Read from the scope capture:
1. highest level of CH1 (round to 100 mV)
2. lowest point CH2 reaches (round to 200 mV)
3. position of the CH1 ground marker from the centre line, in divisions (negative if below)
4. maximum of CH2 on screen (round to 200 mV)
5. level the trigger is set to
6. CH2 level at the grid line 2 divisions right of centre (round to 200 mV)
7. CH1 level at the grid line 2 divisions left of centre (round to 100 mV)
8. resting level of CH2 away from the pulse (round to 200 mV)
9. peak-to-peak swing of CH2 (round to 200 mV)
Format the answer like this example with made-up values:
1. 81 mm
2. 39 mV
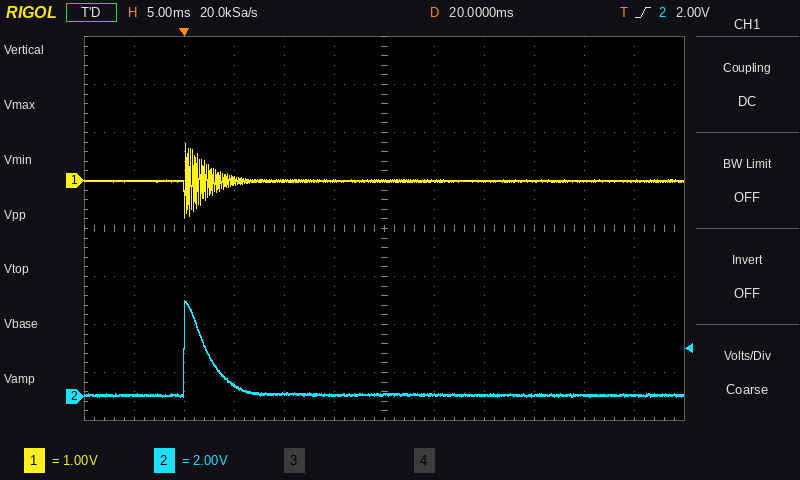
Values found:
1. 800 mV
2. 0.0 V
3. +1.0 div
4. 4.0 V
5. 2.00 V
6. 0.0 V
7. 0.0 V
8. 0.0 V
9. 4.0 V
